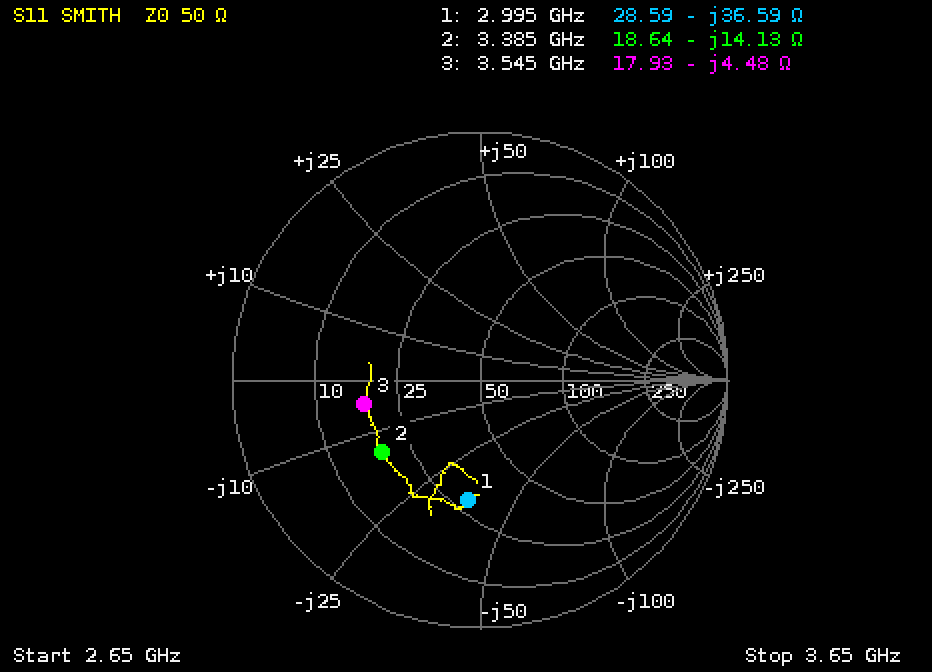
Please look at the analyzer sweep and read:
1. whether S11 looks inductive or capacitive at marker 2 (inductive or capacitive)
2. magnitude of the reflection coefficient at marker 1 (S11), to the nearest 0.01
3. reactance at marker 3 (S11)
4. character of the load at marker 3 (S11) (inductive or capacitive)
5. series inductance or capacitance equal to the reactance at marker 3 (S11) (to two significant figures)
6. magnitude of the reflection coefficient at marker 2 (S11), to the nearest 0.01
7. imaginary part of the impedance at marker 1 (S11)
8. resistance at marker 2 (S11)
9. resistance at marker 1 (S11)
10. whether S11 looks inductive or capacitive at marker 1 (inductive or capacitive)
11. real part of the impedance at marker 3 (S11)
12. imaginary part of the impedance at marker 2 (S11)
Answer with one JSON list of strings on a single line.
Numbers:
["capacitive", "0.49", "-4.48 Ω", "capacitive", "10 pF", "0.49", "-36.59 Ω", "18.64 Ω", "28.59 Ω", "capacitive", "17.93 Ω", "-14.13 Ω"]
